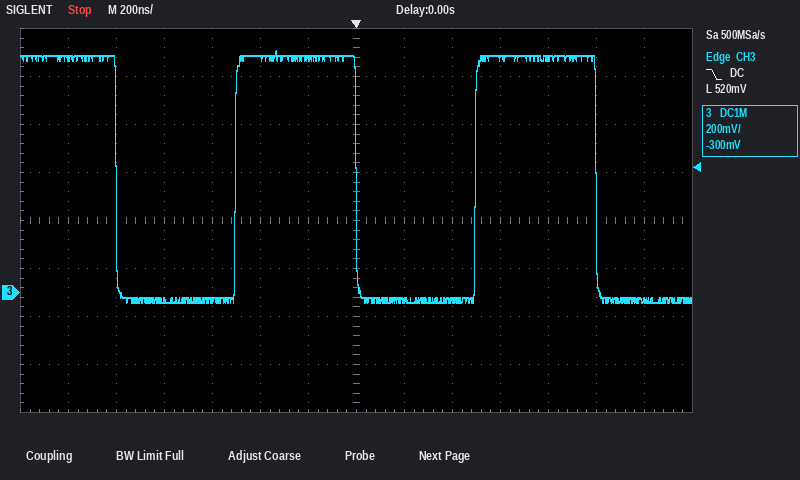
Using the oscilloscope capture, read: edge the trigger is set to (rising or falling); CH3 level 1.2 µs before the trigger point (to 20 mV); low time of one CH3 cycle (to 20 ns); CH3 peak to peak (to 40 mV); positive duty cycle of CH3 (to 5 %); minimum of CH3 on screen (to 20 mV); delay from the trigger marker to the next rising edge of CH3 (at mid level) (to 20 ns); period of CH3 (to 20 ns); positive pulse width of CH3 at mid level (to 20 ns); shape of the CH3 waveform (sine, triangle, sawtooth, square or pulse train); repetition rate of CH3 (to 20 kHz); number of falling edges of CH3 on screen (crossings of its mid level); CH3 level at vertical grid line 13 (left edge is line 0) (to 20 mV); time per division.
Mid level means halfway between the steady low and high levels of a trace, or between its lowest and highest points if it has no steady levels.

falling
980 mV
500 ns
1.04 V
50 %
-40 mV
500 ns
1.00 µs
500 ns
square
1.00 MHz
3
-40 mV
200 ns
